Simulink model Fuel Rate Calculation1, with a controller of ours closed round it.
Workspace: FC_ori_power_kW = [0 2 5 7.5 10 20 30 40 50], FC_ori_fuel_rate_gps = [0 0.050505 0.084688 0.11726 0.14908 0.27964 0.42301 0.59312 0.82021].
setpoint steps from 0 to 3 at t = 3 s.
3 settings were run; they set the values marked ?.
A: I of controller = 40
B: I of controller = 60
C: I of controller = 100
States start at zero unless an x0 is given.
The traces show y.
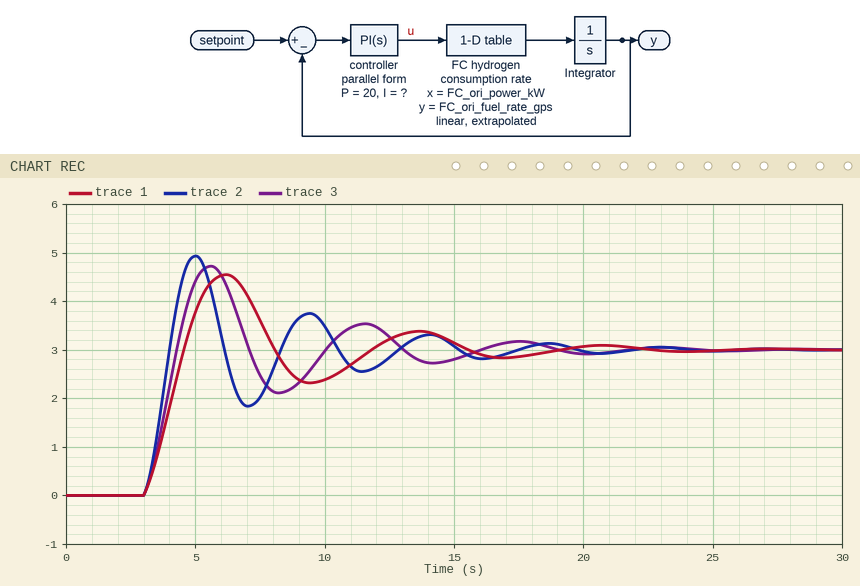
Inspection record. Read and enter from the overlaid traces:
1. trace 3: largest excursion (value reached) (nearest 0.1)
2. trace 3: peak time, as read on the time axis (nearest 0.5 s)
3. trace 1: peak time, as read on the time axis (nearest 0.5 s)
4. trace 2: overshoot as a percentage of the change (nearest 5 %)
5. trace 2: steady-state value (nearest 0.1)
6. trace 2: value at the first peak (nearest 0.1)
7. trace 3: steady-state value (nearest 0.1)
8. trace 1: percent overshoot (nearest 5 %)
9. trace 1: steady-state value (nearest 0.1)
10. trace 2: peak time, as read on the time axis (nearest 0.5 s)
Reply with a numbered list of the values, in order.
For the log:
1. 4.7
2. 5.5 s
3. 6.0 s
4. 65 %
5. 3.0
6. 4.9
7. 3.0
8. 50 %
9. 3.0
10. 5.0 s
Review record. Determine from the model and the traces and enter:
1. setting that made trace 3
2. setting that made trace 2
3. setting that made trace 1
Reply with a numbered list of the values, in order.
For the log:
1. B
2. C
3. A
